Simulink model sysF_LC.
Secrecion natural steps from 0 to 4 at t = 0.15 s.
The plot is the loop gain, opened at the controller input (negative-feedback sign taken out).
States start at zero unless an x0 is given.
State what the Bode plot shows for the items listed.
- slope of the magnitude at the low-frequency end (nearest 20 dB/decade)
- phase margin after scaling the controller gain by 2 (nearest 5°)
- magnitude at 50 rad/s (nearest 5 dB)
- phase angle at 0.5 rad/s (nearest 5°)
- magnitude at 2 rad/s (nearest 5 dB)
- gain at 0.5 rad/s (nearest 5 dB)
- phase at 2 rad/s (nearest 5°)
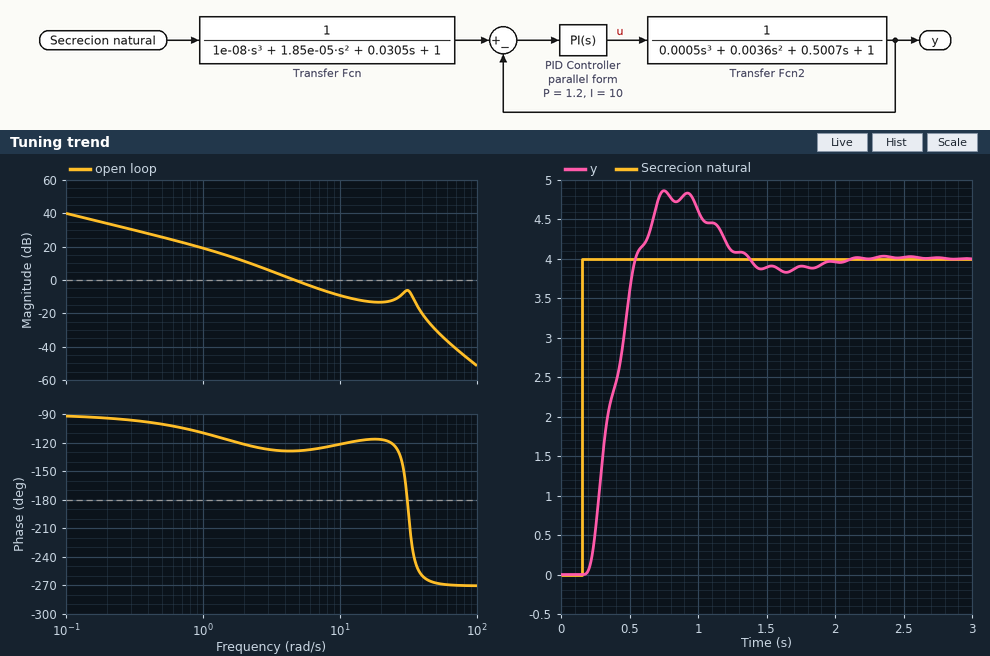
-20 dB/decade
55°
-30 dB
-100°
10 dB
25 dB
-120°
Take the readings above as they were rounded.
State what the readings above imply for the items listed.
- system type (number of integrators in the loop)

1
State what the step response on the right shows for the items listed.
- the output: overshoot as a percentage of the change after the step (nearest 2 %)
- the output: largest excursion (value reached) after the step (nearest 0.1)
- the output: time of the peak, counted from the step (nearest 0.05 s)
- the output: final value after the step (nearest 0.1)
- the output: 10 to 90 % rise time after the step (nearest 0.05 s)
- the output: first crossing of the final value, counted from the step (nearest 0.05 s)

22 %
4.9
0.60 s
4.0
0.25 s
0.40 s
